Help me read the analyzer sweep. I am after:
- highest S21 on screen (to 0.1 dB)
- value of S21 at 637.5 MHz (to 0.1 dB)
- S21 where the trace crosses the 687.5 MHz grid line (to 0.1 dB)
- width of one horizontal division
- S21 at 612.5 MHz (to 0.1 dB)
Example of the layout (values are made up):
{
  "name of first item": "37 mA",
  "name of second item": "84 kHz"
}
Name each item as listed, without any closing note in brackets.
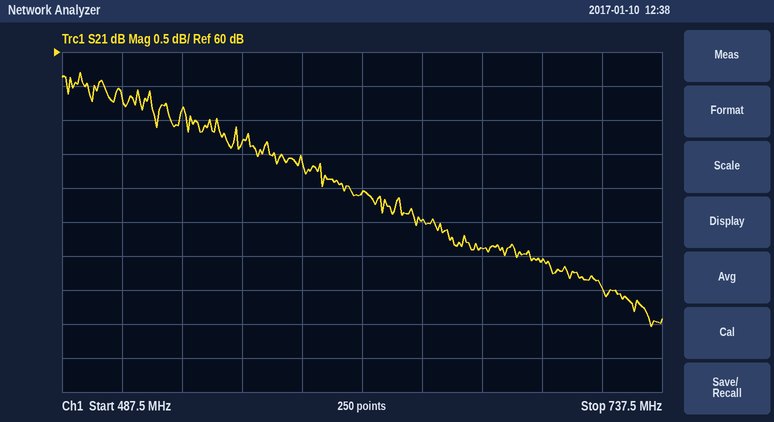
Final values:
{
  "highest S21 on screen": "59.7 dB",
  "value of S21 at 637.5 MHz": "57.5 dB",
  "S21 where the trace crosses the 687.5 MHz grid line": "56.9 dB",
  "width of one horizontal division": "25 MHz",
  "S21 at 612.5 MHz": "57.9 dB"
}
